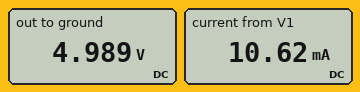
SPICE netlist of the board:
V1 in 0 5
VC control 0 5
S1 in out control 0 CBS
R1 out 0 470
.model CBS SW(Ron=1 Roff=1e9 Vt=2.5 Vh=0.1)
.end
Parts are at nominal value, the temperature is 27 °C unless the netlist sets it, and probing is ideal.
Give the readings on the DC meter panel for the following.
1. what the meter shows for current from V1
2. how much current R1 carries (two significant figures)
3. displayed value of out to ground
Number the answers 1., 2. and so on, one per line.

1. 10.62 mA
2. 11 mA
3. 4.989 V
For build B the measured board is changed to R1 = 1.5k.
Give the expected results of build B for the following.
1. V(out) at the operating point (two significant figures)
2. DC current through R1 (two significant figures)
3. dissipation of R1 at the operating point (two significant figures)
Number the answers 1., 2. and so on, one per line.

1. 5.0 V
2. 3.3 mA
3. 17 mW
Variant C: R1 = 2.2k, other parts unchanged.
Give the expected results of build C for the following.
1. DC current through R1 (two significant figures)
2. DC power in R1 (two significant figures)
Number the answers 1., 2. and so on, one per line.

1. 2.3 mA
2. 11 mW
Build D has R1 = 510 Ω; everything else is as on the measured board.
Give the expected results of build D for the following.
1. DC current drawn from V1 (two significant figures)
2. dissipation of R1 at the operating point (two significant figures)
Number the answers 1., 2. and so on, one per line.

1. 9.8 mA
2. 49 mW
